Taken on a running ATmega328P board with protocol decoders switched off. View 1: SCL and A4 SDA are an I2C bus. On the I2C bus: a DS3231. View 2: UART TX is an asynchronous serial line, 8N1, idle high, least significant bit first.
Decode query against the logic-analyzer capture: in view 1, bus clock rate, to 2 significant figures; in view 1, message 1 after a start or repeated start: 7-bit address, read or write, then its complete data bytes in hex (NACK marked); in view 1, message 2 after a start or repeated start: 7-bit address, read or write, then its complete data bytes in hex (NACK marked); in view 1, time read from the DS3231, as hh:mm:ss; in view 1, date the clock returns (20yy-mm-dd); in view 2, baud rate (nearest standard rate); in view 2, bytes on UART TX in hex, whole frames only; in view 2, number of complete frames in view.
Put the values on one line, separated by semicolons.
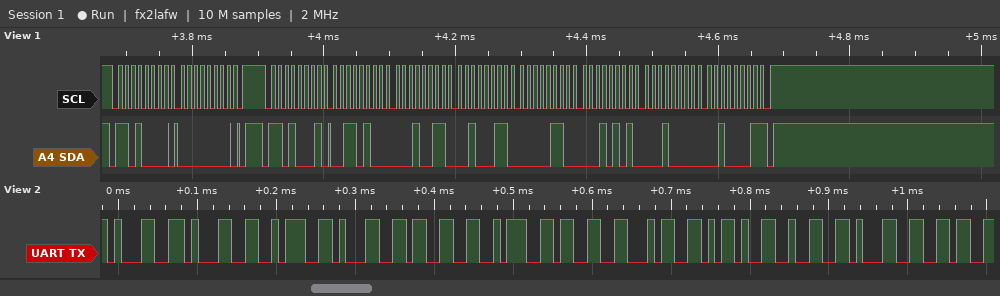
100 kHz; 0x68 write: 00; 0x68 read: 34 13 23 06 15 10 21 NACK; 23:13:34; 2021-10-15; 115200 baud; 0x31 0x31 0x3A 0x31 0x33 0x3A 0x33 0x34 0x2D 0x32 0x31 0x36; 12
